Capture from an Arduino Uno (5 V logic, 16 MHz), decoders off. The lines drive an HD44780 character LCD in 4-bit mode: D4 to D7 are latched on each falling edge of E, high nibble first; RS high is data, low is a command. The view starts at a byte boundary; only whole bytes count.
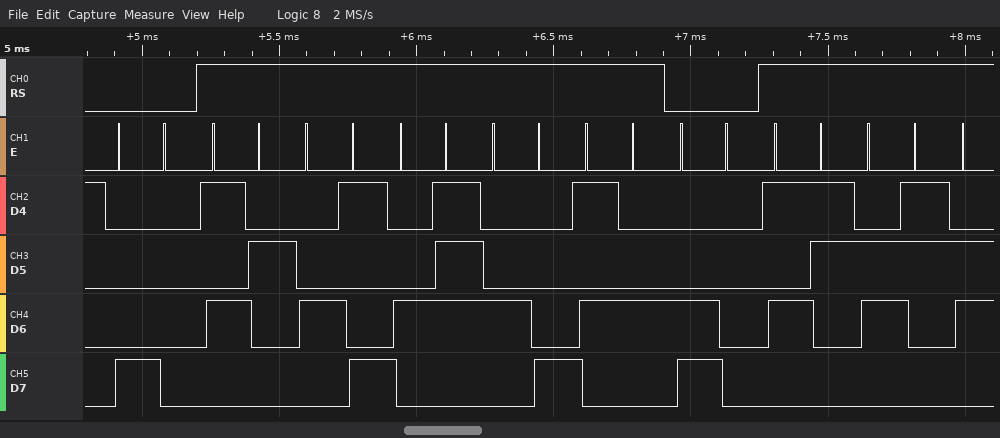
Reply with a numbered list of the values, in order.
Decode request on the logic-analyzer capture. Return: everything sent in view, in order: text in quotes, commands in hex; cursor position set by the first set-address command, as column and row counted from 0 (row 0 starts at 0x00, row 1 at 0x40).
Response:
1. 0x80 "RIGHT" 0xC0 "Sc"
2. column 0, row 0
